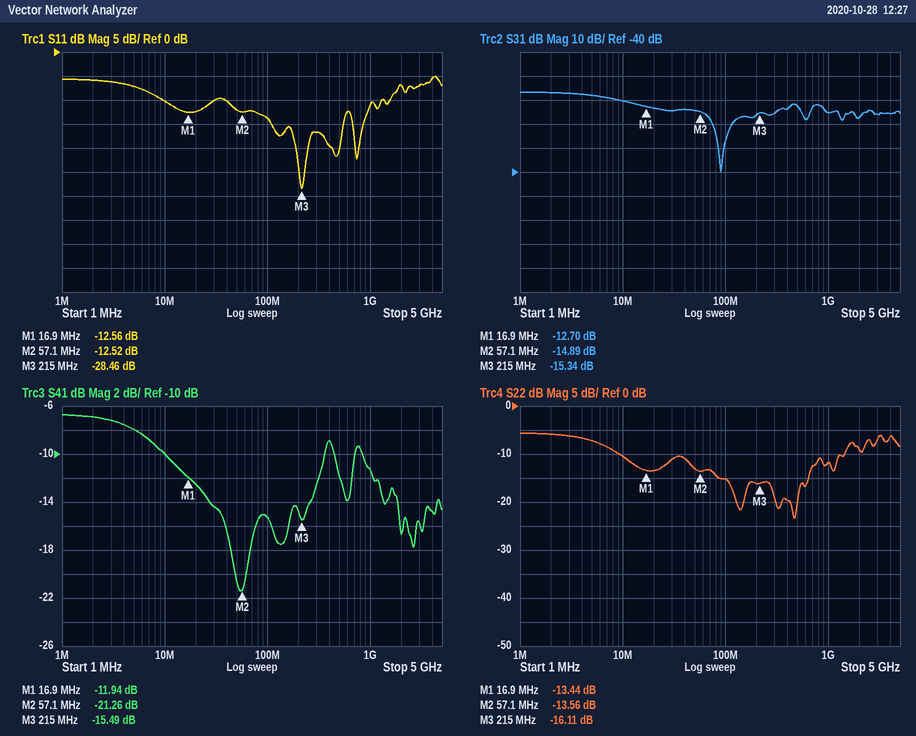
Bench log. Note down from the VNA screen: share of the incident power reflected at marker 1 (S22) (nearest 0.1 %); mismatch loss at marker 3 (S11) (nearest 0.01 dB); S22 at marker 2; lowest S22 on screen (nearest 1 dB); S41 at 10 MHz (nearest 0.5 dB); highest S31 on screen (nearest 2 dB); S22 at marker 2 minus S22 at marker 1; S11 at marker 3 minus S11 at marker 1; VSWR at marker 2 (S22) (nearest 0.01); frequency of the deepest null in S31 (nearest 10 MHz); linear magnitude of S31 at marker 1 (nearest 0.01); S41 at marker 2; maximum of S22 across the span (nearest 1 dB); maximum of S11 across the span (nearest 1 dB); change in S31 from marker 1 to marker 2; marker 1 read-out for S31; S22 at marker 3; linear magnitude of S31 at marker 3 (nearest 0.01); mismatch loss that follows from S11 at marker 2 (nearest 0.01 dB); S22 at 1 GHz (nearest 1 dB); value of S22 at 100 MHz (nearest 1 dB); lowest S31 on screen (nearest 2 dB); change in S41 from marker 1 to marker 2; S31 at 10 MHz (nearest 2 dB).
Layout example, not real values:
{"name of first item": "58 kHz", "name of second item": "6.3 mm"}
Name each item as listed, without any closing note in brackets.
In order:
{"share of the incident power reflected at marker 1 (S22)": "4.5 %", "mismatch loss at marker 3 (S11)": "0.01 dB", "S22 at marker 2": "-13.56 dB", "lowest S22 on screen": "-23 dB", "S41 at 10 MHz": "-10.0 dB", "highest S31 on screen": "-6 dB", "S22 at marker 2 minus S22 at marker 1": "-0.12 dB", "S11 at marker 3 minus S11 at marker 1": "-15.90 dB", "VSWR at marker 2 (S22)": "1.53", "frequency of the deepest null in S31": "90 MHz", "linear magnitude of S31 at marker 1": "0.23", "S41 at marker 2": "-21.26 dB", "maximum of S22 across the span": "-6 dB", "maximum of S11 across the span": "-5 dB", "change in S31 from marker 1 to marker 2": "-2.19 dB", "marker 1 read-out for S31": "-12.70 dB", "S22 at marker 3": "-16.11 dB", "linear magnitude of S31 at marker 3": "0.17", "mismatch loss that follows from S11 at marker 2": "0.25 dB", "S22 at 1 GHz": "-12 dB", "value of S22 at 100 MHz": "-15 dB", "lowest S31 on screen": "-40 dB", "change in S41 from marker 1 to marker 2": "-9.32 dB", "S31 at 10 MHz": "-10 dB"}
